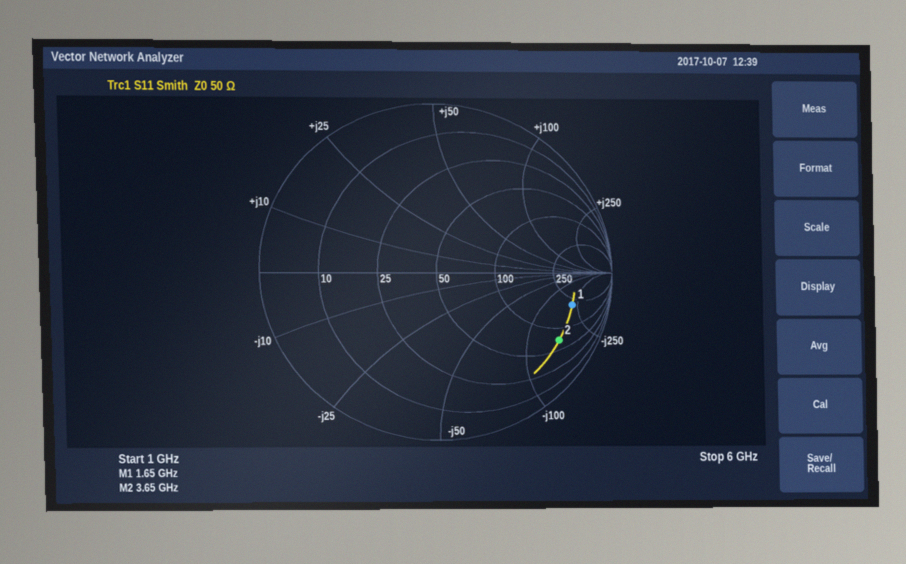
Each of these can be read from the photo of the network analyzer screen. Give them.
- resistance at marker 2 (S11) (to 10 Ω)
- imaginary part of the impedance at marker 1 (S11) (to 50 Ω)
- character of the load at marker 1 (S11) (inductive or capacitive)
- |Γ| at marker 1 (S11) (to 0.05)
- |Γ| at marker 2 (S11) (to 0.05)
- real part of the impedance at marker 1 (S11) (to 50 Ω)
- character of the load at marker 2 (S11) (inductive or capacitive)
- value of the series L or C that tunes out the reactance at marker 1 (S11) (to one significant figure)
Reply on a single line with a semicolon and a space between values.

70 Ω; -200 Ω; capacitive; 0.80; 0.80; 200 Ω; capacitive; 20 nH
